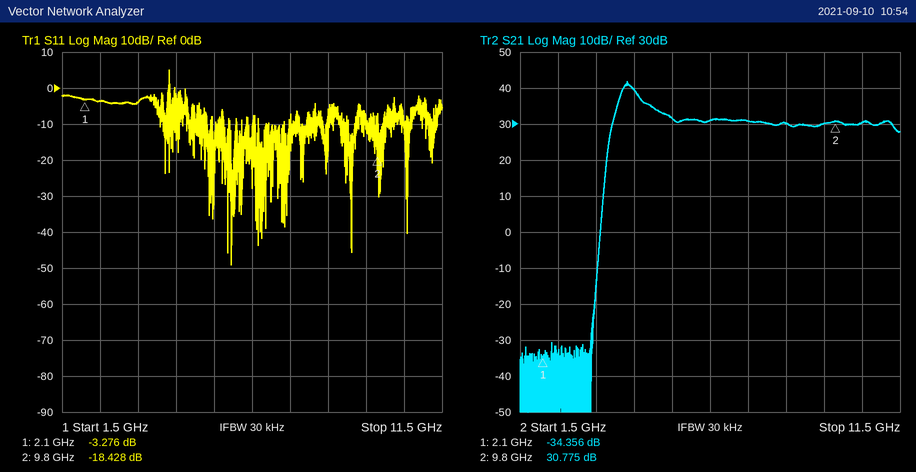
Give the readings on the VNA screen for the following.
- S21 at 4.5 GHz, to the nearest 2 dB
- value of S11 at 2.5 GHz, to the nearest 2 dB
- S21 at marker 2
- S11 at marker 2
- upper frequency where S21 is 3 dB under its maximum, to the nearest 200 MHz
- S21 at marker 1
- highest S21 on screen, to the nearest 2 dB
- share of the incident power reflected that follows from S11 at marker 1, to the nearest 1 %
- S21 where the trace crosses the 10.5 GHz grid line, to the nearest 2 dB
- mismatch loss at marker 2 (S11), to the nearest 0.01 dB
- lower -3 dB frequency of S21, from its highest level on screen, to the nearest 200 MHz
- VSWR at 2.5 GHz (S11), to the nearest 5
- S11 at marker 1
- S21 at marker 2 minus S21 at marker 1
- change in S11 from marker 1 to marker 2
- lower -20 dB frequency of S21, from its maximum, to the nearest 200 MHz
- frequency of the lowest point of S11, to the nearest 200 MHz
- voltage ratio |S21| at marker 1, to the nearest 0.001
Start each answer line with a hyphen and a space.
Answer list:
- 40 dB
- -4 dB
- 30.775 dB
- -18.428 dB
- 4.6 GHz
- -34.356 dB
- 42 dB
- 47 %
- 30 dB
- 0.06 dB
- 4.2 GHz
- 5
- -3.276 dB
- 65.131 dB
- -15.152 dB
- 3.8 GHz
- 6.0 GHz
- 0.019
